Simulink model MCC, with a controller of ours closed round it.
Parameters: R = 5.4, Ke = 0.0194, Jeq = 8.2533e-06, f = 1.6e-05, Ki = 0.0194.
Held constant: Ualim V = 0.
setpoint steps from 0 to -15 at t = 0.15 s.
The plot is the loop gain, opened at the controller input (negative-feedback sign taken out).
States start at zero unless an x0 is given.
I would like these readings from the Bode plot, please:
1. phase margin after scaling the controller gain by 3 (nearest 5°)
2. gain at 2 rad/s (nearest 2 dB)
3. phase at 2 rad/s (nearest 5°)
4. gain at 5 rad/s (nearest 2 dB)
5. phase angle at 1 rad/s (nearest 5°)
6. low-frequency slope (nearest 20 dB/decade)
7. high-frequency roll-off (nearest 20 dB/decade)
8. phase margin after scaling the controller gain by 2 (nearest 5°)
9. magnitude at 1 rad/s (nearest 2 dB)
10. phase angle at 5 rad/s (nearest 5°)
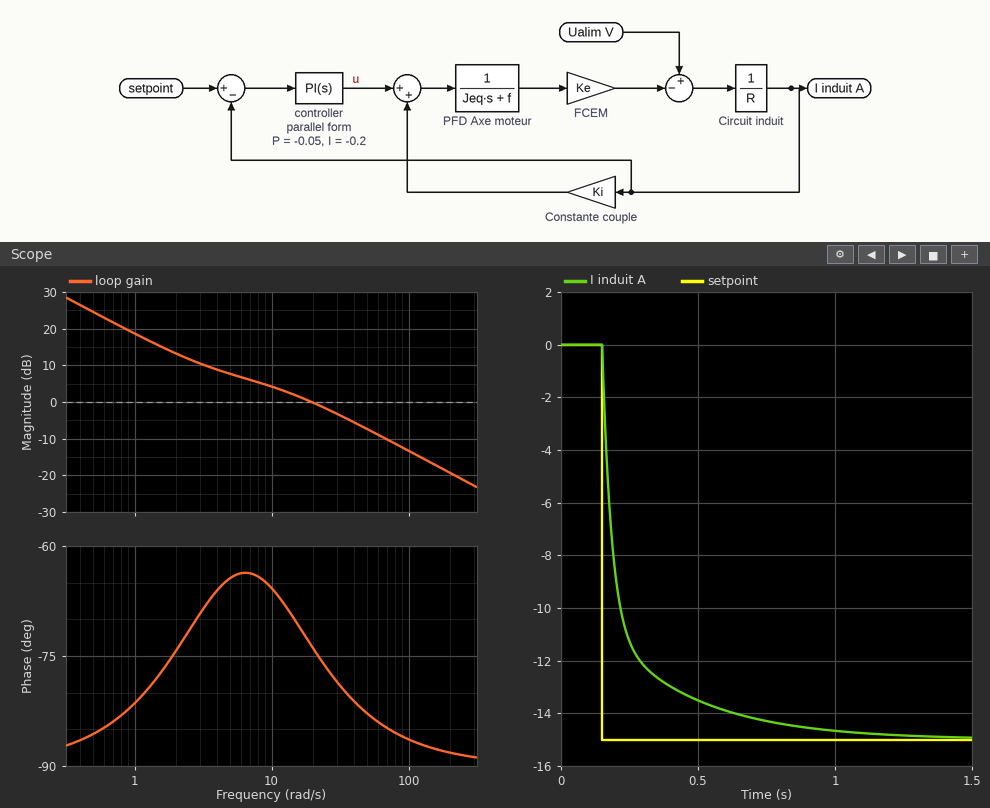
95°
14 dB
-75°
8 dB
-80°
-20 dB/decade
-20 dB/decade
100°
18 dB
-65°
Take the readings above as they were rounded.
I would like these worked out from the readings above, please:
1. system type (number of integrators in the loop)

1
